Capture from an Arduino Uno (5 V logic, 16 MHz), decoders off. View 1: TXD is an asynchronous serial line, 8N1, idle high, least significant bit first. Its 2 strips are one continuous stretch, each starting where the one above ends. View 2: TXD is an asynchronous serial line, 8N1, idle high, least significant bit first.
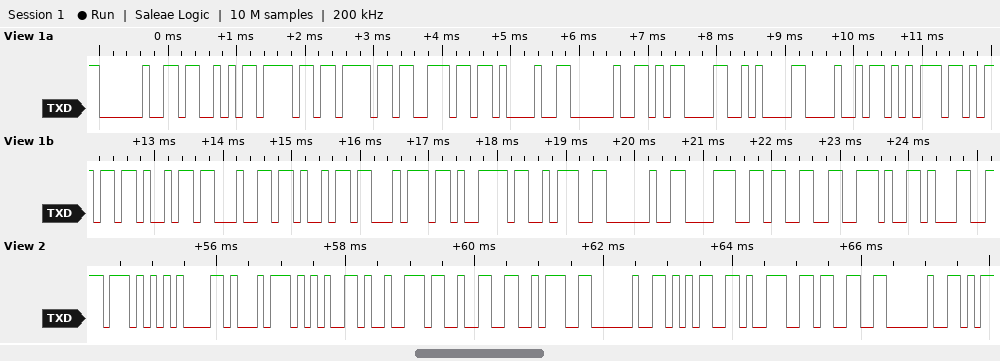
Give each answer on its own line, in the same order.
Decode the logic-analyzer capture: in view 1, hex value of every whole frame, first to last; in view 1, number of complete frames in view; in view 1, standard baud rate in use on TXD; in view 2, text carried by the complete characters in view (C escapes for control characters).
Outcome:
20 53 6F 6F 6E 21 20 0D 0A 48 75 6D 69 64 69 74 79 3A 20 38 33 2E 31
23
9600 baud
"Water2: 593 "
